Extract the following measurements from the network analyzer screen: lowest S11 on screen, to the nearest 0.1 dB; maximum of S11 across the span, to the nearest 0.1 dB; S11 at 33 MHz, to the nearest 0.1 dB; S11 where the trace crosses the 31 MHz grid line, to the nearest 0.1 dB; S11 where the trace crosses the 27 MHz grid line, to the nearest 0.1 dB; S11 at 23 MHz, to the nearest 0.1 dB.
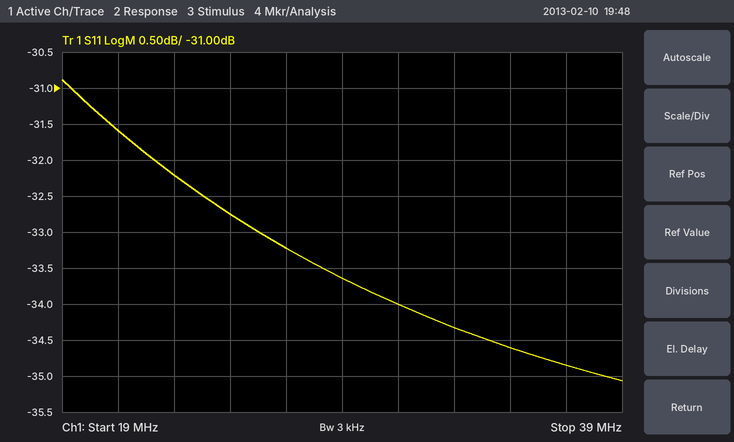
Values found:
-35.1 dB
-30.9 dB
-34.3 dB
-34.0 dB
-33.2 dB
-32.2 dB
